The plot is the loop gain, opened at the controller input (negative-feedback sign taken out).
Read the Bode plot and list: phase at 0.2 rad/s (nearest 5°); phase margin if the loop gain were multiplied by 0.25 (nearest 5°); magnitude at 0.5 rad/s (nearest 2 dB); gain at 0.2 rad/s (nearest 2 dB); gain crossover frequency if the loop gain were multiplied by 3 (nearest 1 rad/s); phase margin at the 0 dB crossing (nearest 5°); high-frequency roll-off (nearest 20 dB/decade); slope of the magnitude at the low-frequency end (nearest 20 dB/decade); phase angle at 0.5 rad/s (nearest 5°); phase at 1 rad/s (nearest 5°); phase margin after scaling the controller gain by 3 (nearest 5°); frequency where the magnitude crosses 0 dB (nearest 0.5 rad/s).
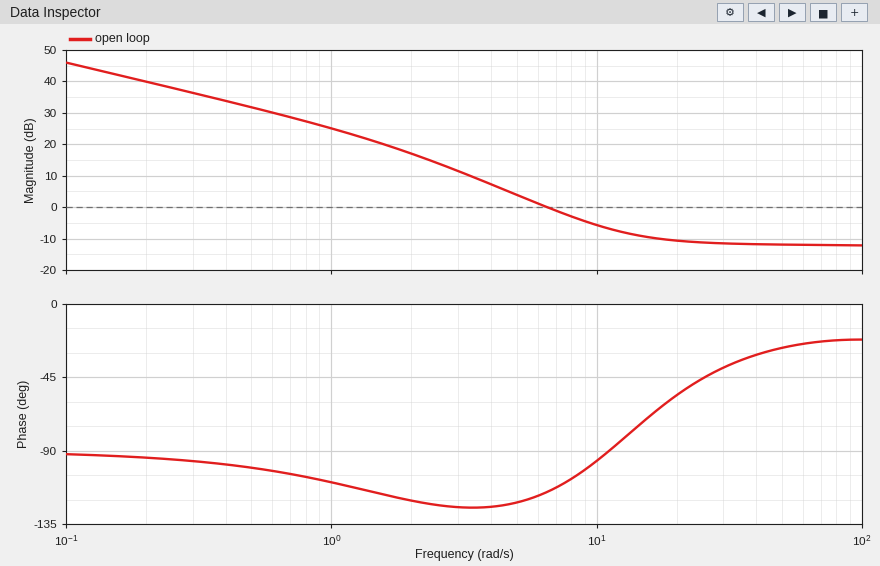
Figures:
-95°
55°
32 dB
40 dB
16 rad/s
65°
0 dB/decade
-20 dB/decade
-100°
-110°
110°
6.5 rad/s
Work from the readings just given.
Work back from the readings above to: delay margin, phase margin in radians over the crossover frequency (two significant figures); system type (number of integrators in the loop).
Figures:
0.17 s
1
